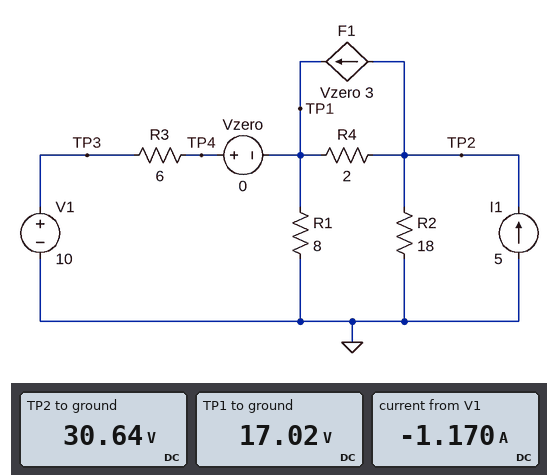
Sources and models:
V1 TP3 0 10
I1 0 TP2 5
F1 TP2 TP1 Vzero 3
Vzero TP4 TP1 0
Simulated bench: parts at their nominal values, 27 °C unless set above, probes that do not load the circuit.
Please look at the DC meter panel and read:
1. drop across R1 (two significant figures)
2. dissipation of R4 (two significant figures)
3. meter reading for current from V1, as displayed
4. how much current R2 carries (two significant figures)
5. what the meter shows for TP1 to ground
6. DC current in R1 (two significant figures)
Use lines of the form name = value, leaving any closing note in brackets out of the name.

drop across R1 = 17 V
dissipation of R4 = 93 W
meter reading for current from V1, as displayed = -1.170 A
how much current R2 carries = 1.7 A
what the meter shows for TP1 to ground = 17.02 V
DC current in R1 = 2.1 A
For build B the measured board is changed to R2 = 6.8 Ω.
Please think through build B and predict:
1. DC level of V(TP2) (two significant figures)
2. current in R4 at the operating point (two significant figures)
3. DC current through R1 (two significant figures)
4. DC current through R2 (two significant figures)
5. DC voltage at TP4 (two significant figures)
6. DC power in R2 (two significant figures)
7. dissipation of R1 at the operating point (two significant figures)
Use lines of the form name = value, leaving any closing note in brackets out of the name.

DC level of V(TP2) = 20 V
current in R4 at the operating point = 3.5 A
DC current through R1 = 1.6 A
DC current through R2 = 2.9 A
DC voltage at TP4 = 13 V
DC power in R2 = 58 W
dissipation of R1 at the operating point = 21 W
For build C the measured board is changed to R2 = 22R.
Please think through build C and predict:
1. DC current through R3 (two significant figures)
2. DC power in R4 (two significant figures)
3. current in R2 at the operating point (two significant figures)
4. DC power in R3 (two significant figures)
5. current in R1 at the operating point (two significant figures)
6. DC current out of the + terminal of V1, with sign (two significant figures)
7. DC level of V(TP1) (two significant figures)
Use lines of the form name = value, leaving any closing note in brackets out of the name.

DC current through R3 = 1.3 A
DC power in R4 = 110 W
current in R2 at the operating point = 1.5 A
DC power in R3 = 10 W
current in R1 at the operating point = 2.2 A
DC current out of the + terminal of V1, with sign = -1.3 A
DC level of V(TP1) = 18 V
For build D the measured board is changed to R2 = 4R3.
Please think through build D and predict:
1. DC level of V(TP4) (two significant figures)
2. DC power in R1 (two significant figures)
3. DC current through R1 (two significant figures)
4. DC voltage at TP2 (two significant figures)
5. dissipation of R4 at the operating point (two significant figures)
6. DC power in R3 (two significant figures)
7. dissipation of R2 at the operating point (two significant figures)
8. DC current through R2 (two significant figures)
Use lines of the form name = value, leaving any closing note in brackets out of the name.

DC level of V(TP4) = 11 V
DC power in R1 = 15 W
DC current through R1 = 1.4 A
DC voltage at TP2 = 15 V
dissipation of R4 at the operating point = 8.0 W
DC power in R3 = 150 mW
dissipation of R2 at the operating point = 52 W
DC current through R2 = 3.5 A
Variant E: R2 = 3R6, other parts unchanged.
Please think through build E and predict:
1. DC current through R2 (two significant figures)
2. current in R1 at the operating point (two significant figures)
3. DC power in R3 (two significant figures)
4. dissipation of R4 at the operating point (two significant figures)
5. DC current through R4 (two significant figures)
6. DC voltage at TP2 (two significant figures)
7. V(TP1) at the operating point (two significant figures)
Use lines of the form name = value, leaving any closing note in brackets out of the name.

DC current through R2 = 3.7 A
current in R1 at the operating point = 1.3 A
DC power in R3 = 13 mW
dissipation of R4 at the operating point = 4.3 W
DC current through R4 = 1.5 A
DC voltage at TP2 = 13 V
V(TP1) at the operating point = 10 V
